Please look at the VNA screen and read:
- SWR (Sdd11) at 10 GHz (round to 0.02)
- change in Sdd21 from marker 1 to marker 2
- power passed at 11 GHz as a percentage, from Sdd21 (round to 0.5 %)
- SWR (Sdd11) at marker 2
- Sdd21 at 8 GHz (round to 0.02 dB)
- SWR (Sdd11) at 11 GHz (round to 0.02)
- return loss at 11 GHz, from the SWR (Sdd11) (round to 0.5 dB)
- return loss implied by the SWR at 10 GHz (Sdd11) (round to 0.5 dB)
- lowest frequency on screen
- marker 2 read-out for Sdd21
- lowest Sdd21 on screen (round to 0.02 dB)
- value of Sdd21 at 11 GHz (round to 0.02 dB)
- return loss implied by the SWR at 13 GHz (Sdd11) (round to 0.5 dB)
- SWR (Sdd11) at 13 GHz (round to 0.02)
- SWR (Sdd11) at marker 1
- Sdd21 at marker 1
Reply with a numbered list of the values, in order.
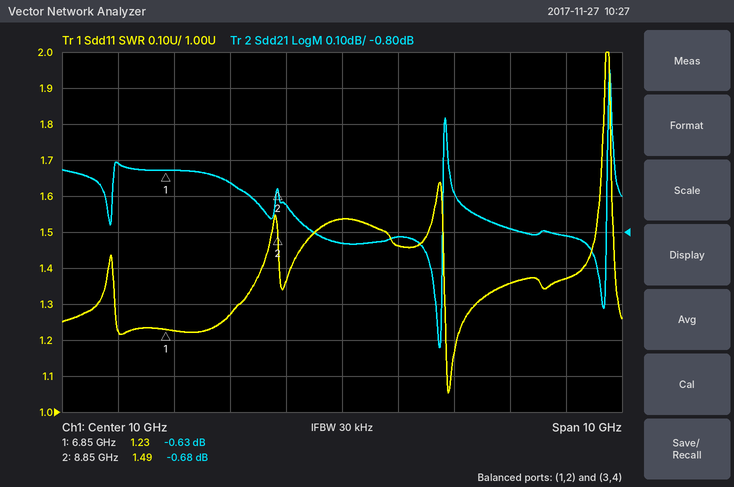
1. 1.54
2. -0.05 dB
3. 83.0 %
4. 1.49
5. -0.66 dB
6. 1.46
7. 14.5 dB
8. 13.5 dB
9. 5 GHz
10. -0.68 dB
11. -1.12 dB
12. -0.82 dB
13. 16.5 dB
14. 1.36
15. 1.23
16. -0.63 dB
